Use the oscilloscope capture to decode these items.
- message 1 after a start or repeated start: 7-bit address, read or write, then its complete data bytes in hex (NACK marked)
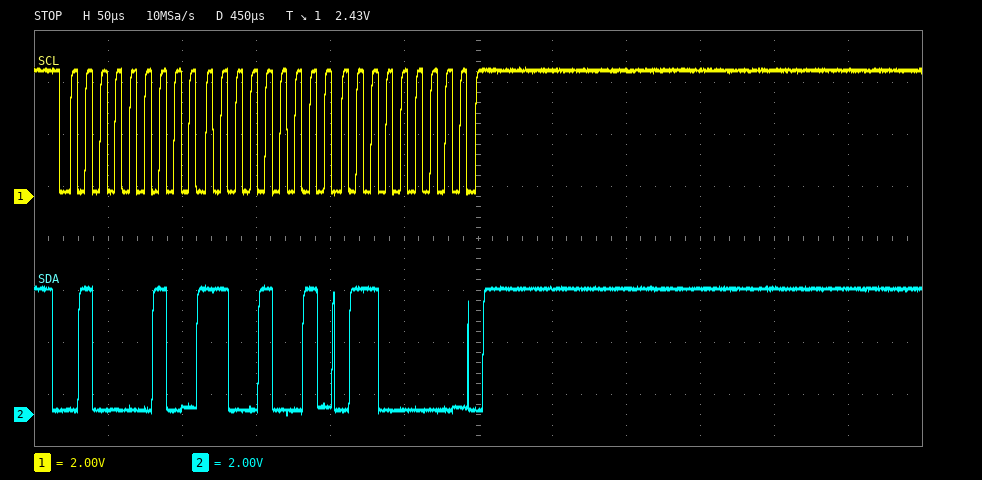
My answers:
0x21 write: C9 60
